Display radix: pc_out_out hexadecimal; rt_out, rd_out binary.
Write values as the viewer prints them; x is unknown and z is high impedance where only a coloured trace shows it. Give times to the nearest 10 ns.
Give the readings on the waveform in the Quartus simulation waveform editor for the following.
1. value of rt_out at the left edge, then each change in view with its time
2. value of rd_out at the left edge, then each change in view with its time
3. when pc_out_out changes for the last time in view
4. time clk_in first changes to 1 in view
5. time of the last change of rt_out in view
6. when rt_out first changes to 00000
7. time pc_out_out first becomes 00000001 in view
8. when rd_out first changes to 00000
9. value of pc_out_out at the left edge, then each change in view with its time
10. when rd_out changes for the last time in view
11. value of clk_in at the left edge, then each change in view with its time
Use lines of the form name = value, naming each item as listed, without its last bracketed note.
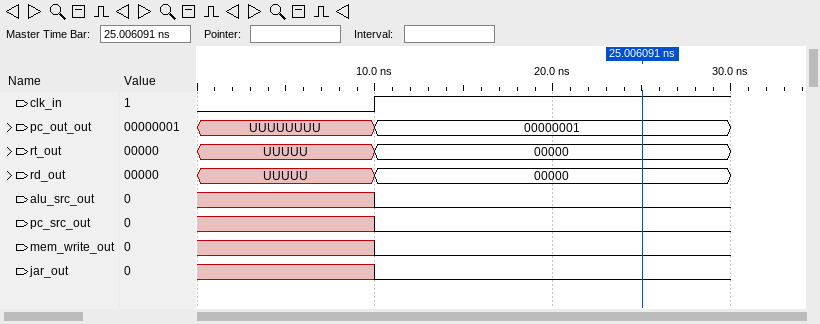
value of rt_out at the left edge, then each change in view with its time = UUUUU, 00000 at 10 ns
value of rd_out at the left edge, then each change in view with its time = UUUUU, 00000 at 10 ns
when pc_out_out changes for the last time in view = 10 ns
time clk_in first changes to 1 in view = 10 ns
time of the last change of rt_out in view = 10 ns
when rt_out first changes to 00000 = 10 ns
time pc_out_out first becomes 00000001 in view = 10 ns
when rd_out first changes to 00000 = 10 ns
value of pc_out_out at the left edge, then each change in view with its time = UUUUUUUU, 00000001 at 10 ns
when rd_out changes for the last time in view = 10 ns
value of clk_in at the left edge, then each change in view with its time = 0, 1 at 10 ns
